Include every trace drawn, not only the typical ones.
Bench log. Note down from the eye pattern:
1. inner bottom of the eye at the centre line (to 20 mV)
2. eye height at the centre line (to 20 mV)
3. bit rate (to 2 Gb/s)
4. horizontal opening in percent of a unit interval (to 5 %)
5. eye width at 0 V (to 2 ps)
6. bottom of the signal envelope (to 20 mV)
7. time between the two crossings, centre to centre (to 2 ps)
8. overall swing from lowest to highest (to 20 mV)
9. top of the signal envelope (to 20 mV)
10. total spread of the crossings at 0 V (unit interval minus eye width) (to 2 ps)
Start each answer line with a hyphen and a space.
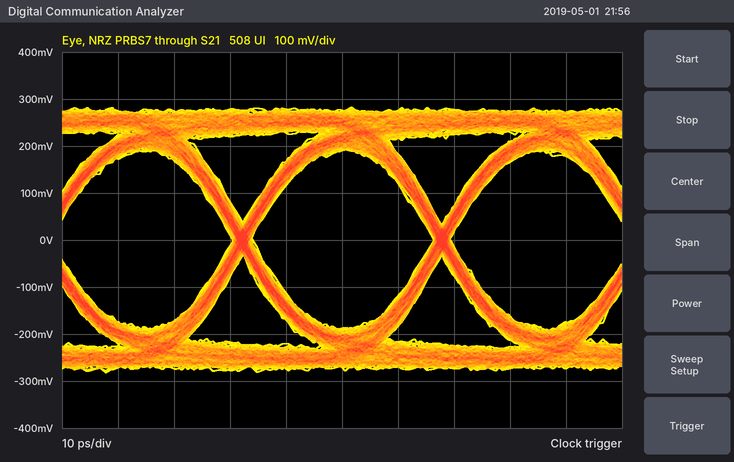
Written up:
- -180 mV
- 380 mV
- 28 Gb/s
- 90 %
- 32 ps
- -280 mV
- 36 ps
- 560 mV
- 280 mV
- 4 ps
